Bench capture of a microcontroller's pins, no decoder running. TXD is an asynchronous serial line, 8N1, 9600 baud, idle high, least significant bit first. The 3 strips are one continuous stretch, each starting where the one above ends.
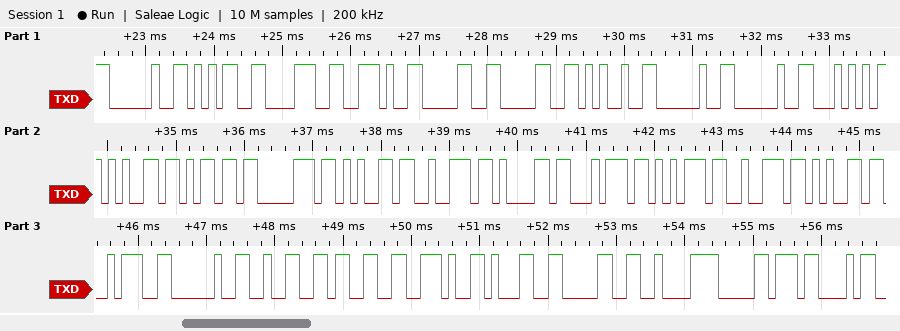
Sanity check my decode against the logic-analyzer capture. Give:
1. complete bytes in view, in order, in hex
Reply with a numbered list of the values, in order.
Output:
1. 20 35 38 2E 30 30 25 20 20 54 65 6D 70 65 72 61 74 75 72 65 3A 20 32 33 2E 31 30 C2 B0 43
